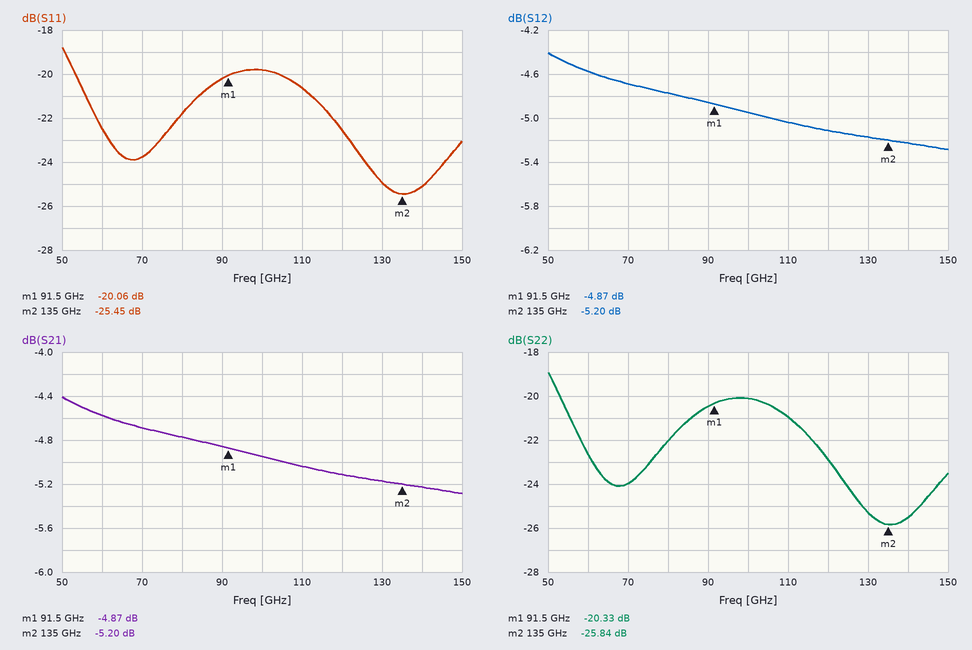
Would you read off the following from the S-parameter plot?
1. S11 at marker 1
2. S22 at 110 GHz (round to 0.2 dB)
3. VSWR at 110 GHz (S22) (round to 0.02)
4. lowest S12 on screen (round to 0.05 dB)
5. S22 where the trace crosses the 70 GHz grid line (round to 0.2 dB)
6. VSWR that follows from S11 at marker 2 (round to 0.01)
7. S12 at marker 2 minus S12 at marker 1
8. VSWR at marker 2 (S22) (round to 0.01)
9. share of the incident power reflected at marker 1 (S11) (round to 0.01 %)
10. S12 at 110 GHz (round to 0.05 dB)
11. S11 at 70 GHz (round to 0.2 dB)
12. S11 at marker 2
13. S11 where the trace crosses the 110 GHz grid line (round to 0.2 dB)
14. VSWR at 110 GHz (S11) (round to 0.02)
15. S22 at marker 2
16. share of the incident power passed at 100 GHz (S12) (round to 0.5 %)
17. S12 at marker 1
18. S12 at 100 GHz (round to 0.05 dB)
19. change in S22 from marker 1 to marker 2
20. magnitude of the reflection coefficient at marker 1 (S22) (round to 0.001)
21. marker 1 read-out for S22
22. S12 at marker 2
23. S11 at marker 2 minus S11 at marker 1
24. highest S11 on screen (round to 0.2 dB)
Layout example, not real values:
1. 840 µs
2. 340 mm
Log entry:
1. -20.06 dB
2. -21.0 dB
3. 1.20
4. -5.30 dB
5. -24.0 dB
6. 1.11
7. -0.33 dB
8. 1.11
9. 0.99 %
10. -5.05 dB
11. -23.8 dB
12. -25.45 dB
13. -20.6 dB
14. 1.20
15. -25.84 dB
16. 32.0 %
17. -4.87 dB
18. -4.95 dB
19. -5.51 dB
20. 0.096
21. -20.33 dB
22. -5.20 dB
23. -5.39 dB
24. -18.8 dB
